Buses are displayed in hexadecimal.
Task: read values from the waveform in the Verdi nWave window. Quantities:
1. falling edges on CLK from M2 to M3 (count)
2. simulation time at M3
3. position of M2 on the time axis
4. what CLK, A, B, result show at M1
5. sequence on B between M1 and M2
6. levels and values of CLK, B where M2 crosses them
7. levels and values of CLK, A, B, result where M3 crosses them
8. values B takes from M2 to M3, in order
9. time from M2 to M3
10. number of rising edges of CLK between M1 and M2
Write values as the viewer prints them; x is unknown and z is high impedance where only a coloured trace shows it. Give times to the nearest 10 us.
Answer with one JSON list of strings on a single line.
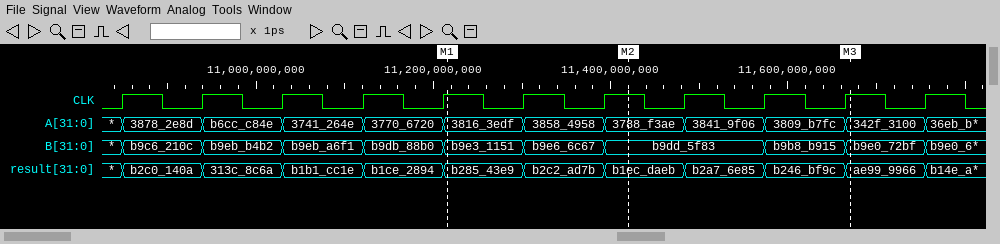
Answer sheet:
["3", "11670 us", "11420 us", "CLK=1, A=3816_3edf, B=b9e3_1151, result=b285_43e9", "b9e3_1151, b9e6_6c67, b9dd_5f83", "CLK=1, B=b9dd_5f83", "CLK=1, A=342f_3100, B=b9e0_72bf, result=ae99_9966", "b9dd_5f83, b9b8_b915, b9e0_72bf", "250 us", "2"]
